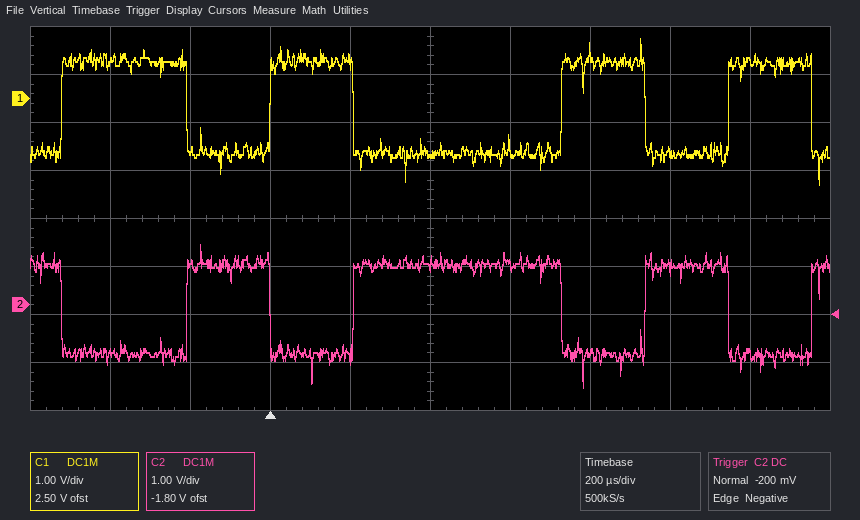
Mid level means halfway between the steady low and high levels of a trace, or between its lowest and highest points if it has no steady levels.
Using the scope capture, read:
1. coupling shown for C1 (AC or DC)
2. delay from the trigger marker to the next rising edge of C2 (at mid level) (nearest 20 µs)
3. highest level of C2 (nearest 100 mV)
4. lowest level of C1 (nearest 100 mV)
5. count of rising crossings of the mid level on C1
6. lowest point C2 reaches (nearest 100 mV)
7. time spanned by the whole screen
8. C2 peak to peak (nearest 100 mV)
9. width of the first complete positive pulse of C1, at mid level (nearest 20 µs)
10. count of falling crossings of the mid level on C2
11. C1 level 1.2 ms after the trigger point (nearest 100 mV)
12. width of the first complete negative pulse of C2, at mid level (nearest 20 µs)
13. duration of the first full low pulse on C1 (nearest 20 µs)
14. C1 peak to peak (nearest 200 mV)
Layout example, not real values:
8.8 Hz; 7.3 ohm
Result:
DC; 200 µs; 1.3 V; -1.8 V; 4; -1.7 V; 2 ms; 3.0 V; 320 µs; 4; 800 mV; 320 µs; 200 µs; 3.0 V
